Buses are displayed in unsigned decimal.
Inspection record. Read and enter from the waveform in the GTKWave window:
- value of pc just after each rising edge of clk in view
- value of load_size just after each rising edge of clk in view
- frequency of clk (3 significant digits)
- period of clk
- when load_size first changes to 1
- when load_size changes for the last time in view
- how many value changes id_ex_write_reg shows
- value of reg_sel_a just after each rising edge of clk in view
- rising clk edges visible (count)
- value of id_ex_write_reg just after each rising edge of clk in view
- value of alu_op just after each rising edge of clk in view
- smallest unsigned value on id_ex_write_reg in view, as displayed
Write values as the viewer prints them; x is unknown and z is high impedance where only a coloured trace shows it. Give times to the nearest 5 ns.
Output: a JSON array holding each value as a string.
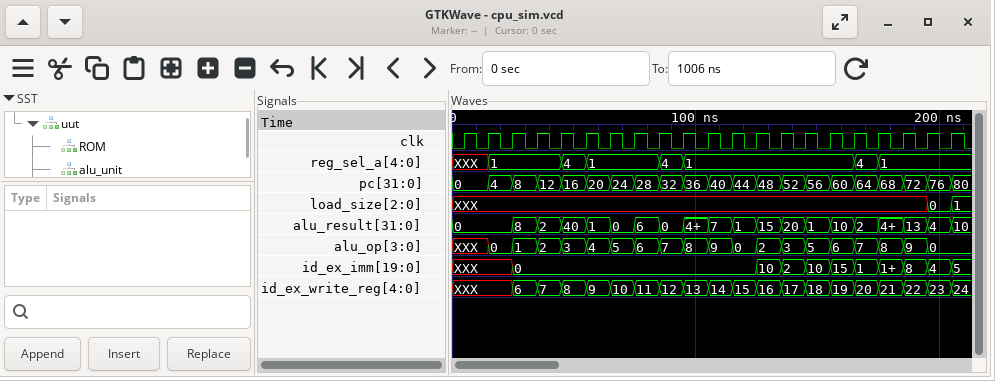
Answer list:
["0, 4, 8, 12, 16, 20, 24, 28, 32, 36, 40, 44, 48, 52, 56, 60, 64, 68, 72, 76, 80", "XXX, XXX, XXX, XXX, XXX, XXX, XXX, XXX, XXX, XXX, XXX, XXX, XXX, XXX, XXX, XXX, XXX, XXX, XXX, 0, 1", "100 MHz", "10 ns", "205 ns", "205 ns", "19", "XXX, 1, 1, 1, 4, 1, 1, 1, 4, 1, 1, 1, 1, 1, 1, 1, 4, 1, 1, 1, 1", "21", "XXX, XXX, 6, 7, 8, 9, 10, 11, 12, 13, 14, 15, 16, 17, 18, 19, 20, 21, 22, 23, 24", "XXX, 0, 1, 2, 3, 4, 5, 6, 7, 8, 9, 0, 2, 3, 5, 6, 7, 8, 9, 0, 0", "6"]
